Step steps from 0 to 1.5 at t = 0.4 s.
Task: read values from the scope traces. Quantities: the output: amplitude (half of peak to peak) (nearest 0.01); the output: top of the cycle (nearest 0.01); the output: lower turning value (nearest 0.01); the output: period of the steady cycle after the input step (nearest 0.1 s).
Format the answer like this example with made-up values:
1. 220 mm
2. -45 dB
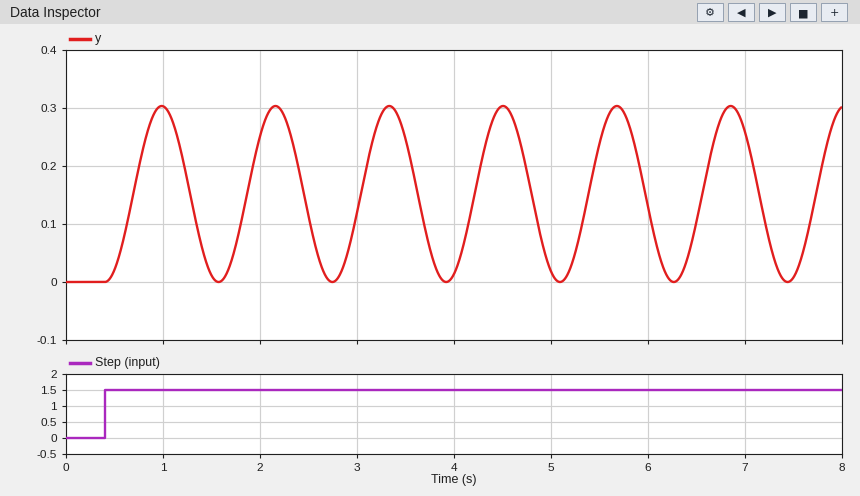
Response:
1. 0.15
2. 0.30
3. 0.00
4. 1.2 s
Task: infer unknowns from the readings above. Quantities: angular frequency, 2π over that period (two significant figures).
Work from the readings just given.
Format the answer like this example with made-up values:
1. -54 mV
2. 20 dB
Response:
1. 5.2 rad/s
